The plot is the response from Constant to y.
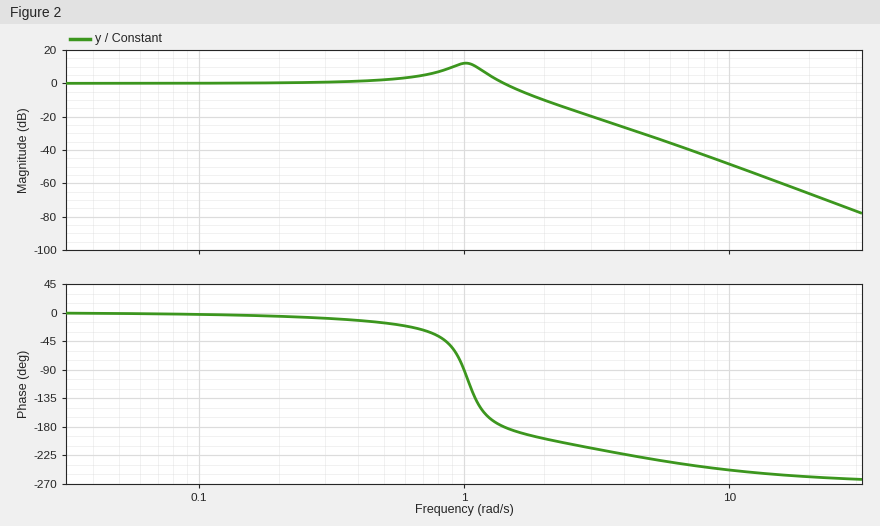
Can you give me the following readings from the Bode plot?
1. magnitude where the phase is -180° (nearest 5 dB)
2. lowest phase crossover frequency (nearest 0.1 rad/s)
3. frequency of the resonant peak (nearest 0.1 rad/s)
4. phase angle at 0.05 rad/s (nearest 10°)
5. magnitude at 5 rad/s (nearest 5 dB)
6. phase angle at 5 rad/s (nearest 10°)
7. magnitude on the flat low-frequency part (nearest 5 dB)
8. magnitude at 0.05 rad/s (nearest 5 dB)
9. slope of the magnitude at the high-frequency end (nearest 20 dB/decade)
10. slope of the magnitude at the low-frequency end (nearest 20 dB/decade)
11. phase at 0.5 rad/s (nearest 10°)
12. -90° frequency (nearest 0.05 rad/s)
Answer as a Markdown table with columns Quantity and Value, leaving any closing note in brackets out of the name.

| Quantity | Value |
|---|---|
| magnitude where the phase is -180° | 0 dB |
| lowest phase crossover frequency | 1.4 rad/s |
| frequency of the resonant peak | 1.0 rad/s |
| phase angle at 0.05 rad/s | 0° |
| magnitude at 5 rad/s | -30 dB |
| phase angle at 5 rad/s | -230° |
| magnitude on the flat low-frequency part | 0 dB |
| magnitude at 0.05 rad/s | 0 dB |
| slope of the magnitude at the high-frequency end | -60 dB/decade |
| slope of the magnitude at the low-frequency end | 0 dB/decade |
| phase at 0.5 rad/s | -20° |
| -90° frequency | 1.00 rad/s |
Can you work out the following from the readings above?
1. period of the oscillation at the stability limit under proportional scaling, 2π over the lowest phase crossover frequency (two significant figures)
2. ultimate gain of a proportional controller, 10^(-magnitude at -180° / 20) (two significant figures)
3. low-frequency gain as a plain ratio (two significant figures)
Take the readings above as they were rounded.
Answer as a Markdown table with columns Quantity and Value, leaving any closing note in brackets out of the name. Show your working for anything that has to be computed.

| Quantity | Value |
|---|---|
| period of the oscillation at the stability limit under proportional scaling, 2π over the lowest phase crossover frequency | 2π / 1.4 = 4.5 s |
| ultimate gain of a proportional controller, 10^(-magnitude at -180° / 20) | 10^(0 / 20) = 1.0 |
| low-frequency gain as a plain ratio | 10^(0 / 20) = 1.0 |
